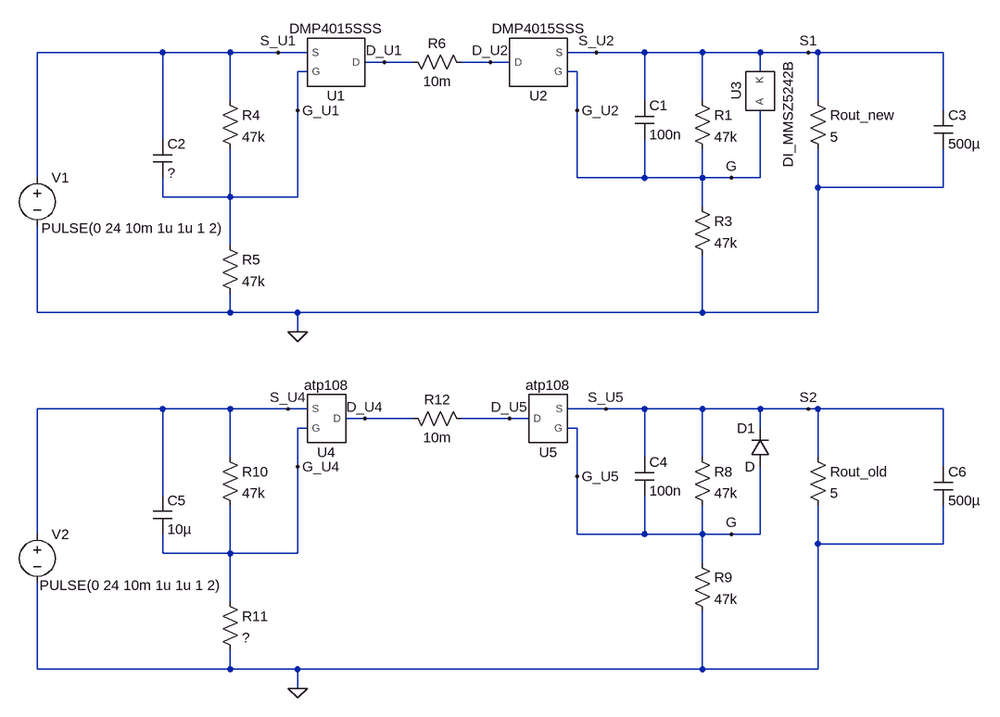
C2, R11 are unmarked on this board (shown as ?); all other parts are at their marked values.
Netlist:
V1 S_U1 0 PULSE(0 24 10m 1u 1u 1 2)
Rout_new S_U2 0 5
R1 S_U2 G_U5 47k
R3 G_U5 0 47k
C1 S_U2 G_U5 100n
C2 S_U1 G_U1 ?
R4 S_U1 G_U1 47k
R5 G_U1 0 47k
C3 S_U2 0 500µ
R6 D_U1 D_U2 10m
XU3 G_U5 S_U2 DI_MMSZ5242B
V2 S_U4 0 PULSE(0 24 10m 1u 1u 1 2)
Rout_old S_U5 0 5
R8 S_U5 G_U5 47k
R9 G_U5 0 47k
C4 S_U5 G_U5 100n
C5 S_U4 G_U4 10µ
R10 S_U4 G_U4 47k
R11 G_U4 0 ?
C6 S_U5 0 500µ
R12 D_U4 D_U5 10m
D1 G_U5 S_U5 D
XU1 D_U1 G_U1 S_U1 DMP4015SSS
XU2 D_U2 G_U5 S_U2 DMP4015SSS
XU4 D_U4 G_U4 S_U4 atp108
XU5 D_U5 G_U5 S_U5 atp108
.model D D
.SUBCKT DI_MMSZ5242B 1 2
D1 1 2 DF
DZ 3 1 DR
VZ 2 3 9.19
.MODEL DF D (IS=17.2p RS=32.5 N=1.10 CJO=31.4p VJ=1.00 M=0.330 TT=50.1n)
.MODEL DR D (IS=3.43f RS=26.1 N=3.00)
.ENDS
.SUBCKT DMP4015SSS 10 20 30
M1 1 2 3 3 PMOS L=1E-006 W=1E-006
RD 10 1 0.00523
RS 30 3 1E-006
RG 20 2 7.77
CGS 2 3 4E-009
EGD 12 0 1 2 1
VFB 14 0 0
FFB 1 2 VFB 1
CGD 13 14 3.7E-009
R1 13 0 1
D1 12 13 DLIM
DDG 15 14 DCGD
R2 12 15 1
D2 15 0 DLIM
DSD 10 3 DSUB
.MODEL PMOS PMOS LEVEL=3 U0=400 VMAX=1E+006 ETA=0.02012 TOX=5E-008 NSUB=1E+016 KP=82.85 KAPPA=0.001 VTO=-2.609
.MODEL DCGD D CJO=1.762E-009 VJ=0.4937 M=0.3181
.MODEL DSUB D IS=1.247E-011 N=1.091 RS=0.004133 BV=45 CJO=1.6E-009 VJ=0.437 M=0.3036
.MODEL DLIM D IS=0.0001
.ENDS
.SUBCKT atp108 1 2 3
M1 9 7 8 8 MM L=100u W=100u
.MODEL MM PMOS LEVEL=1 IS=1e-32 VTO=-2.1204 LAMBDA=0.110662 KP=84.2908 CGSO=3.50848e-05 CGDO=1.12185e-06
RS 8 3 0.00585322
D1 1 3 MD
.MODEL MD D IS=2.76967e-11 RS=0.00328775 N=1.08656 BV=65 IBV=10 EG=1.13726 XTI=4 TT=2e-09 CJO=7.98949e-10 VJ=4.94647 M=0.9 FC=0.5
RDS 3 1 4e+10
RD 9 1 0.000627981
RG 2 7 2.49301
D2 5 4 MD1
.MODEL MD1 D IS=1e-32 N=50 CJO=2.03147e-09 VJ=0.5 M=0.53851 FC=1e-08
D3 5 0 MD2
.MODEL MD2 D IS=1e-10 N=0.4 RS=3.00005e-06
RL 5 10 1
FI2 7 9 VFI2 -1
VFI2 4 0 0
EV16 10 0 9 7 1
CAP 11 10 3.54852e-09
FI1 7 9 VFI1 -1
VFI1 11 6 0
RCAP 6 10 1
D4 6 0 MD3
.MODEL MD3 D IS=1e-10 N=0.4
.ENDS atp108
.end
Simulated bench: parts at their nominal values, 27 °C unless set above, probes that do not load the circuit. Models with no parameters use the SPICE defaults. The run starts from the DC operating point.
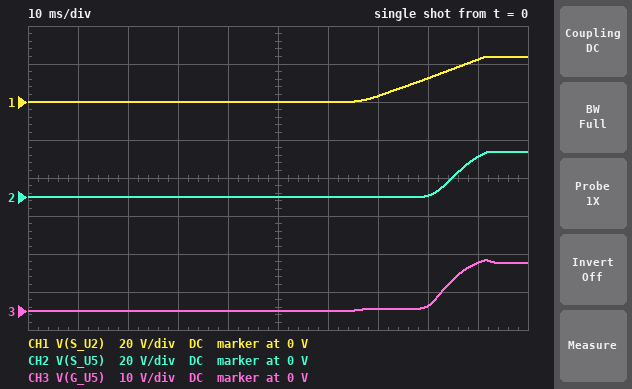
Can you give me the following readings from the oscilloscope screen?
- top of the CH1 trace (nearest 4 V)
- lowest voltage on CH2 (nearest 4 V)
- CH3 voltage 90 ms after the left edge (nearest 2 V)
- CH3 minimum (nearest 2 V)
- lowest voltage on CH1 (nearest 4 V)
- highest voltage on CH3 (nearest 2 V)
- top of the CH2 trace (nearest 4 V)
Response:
24 V
0 V
12 V
0 V
0 V
14 V
24 V
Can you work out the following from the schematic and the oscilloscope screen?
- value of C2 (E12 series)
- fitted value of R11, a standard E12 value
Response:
12 µF
68 kΩ
